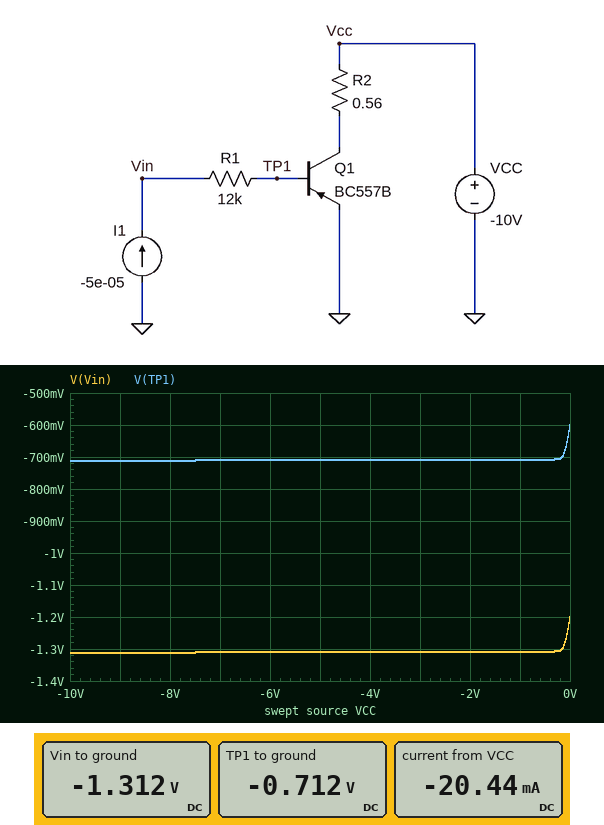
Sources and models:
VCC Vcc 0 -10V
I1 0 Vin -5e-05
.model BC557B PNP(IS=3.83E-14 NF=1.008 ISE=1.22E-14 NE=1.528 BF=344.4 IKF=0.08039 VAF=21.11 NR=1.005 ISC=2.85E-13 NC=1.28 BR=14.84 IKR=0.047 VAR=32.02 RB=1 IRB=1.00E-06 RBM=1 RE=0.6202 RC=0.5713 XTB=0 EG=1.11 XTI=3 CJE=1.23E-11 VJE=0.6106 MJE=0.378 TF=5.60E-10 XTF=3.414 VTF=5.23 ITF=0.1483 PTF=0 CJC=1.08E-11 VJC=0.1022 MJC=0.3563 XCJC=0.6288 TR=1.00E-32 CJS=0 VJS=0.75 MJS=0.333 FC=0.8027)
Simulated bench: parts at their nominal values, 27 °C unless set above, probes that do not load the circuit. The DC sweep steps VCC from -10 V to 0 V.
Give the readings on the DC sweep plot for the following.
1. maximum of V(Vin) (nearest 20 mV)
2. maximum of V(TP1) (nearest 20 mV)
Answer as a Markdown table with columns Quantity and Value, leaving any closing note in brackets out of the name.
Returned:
| Quantity | Value |
|---|---|
| maximum of V(Vin) | -1.20 V |
| maximum of V(TP1) | -600 mV |
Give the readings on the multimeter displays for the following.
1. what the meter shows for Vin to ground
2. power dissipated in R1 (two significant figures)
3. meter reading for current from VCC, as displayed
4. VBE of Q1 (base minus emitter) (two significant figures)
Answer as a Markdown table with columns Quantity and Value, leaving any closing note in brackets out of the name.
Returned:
| Quantity | Value |
|---|---|
| what the meter shows for Vin to ground | -1.312 V |
| power dissipated in R1 | 30 µW |
| meter reading for current from VCC, as displayed | -20.44 mA |
| VBE of Q1 (base minus emitter) | -710 mV |
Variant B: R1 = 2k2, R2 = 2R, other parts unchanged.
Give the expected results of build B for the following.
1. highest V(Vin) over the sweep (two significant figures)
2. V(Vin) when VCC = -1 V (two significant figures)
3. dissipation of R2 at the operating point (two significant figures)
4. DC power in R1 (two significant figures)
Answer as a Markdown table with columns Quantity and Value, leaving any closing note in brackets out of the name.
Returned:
| Quantity | Value |
|---|---|
| highest V(Vin) over the sweep | -710 mV |
| V(Vin) when VCC = -1 V | -820 mV |
| dissipation of R2 at the operating point | 830 µW |
| DC power in R1 | 5.5 µW |
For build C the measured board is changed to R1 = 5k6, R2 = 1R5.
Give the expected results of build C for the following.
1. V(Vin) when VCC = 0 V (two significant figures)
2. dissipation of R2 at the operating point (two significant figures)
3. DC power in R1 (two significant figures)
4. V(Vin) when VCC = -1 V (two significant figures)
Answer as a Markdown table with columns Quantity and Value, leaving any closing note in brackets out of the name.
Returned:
| Quantity | Value |
|---|---|
| V(Vin) when VCC = 0 V | -880 mV |
| dissipation of R2 at the operating point | 630 µW |
| DC power in R1 | 14 µW |
| V(Vin) when VCC = -1 V | -990 mV |
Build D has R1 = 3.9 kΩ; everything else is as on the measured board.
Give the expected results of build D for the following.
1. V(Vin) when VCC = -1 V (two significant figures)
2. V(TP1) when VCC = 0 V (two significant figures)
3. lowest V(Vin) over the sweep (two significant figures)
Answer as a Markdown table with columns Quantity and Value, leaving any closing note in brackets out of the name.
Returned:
| Quantity | Value |
|---|---|
| V(Vin) when VCC = -1 V | -900 mV |
| V(TP1) when VCC = 0 V | -600 mV |
| lowest V(Vin) over the sweep | -910 mV |
